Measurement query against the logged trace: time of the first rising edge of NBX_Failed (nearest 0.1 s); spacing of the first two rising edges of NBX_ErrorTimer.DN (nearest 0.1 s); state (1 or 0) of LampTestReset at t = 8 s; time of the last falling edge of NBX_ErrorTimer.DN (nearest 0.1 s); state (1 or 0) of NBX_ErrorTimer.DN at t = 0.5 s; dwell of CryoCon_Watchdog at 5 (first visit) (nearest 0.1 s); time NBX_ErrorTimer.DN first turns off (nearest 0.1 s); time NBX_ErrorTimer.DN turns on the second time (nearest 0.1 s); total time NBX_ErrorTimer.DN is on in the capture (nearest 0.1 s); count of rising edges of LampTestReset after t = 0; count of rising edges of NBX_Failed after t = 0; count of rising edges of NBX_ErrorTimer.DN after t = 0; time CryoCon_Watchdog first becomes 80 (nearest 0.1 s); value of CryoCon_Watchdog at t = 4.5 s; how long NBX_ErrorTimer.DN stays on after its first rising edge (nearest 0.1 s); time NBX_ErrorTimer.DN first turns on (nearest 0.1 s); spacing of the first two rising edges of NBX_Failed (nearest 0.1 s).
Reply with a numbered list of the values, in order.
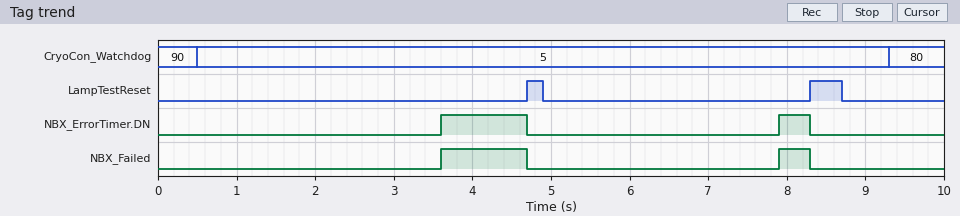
1. 3.6 s
2. 4.3 s
3. 0
4. 8.3 s
5. 0
6. 8.8 s
7. 4.7 s
8. 7.9 s
9. 1.5 s
10. 2
11. 2
12. 2
13. 9.3 s
14. 5
15. 1.1 s
16. 3.6 s
17. 4.3 s
